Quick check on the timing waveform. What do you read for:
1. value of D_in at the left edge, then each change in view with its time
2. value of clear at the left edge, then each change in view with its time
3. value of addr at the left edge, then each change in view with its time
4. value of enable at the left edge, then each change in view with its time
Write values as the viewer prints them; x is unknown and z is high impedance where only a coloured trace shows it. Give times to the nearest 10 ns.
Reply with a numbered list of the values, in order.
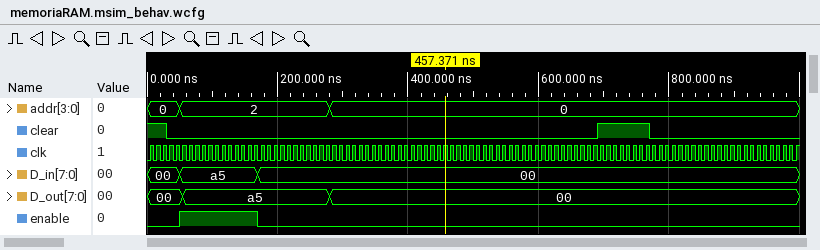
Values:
1. 00, a5 at 50 ns, 00 at 170 ns
2. 1, 0 at 30 ns, 1 at 690 ns, 0 at 770 ns
3. 0, 2 at 50 ns, 0 at 280 ns
4. 0, 1 at 50 ns, 0 at 170 ns
